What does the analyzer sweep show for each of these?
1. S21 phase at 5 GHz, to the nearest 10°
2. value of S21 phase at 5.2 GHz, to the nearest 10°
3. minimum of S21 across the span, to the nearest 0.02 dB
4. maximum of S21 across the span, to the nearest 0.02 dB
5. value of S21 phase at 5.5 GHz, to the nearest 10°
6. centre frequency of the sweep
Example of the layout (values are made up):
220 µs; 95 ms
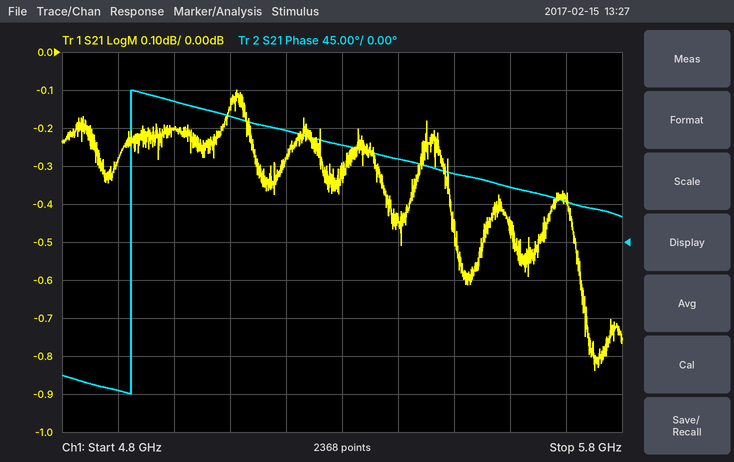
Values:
170°; 130°; -0.84 dB; -0.10 dB; 80°; 5.3 GHz
